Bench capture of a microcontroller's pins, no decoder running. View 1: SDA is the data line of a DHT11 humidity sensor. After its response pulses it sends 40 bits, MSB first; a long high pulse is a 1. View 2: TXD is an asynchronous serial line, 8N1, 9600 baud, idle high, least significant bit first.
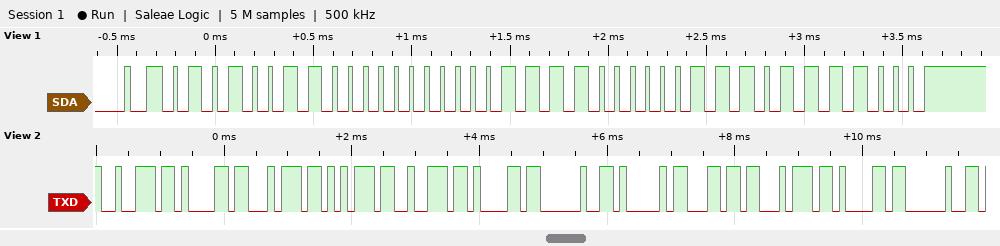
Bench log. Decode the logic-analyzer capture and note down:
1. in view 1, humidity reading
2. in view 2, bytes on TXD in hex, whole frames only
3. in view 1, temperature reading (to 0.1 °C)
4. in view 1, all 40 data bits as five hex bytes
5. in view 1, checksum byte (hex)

83 %
72 61 74 75 72 61 20 41 6C 74 61 20
30.7 °C
53 00 1E 07 78
0x78
